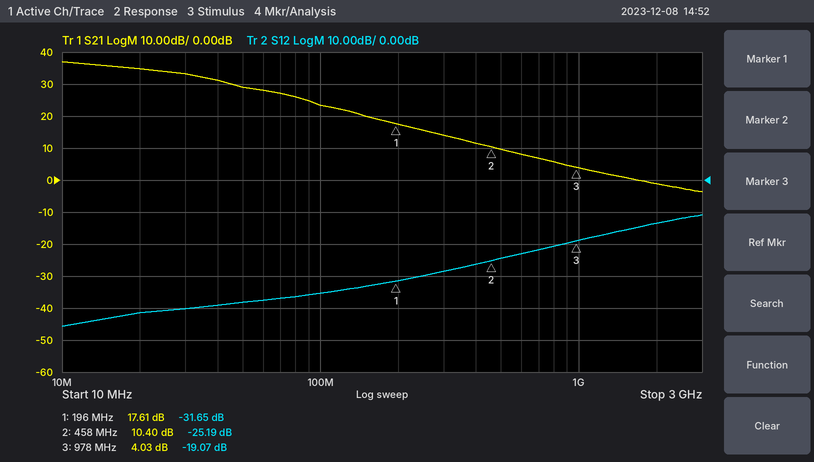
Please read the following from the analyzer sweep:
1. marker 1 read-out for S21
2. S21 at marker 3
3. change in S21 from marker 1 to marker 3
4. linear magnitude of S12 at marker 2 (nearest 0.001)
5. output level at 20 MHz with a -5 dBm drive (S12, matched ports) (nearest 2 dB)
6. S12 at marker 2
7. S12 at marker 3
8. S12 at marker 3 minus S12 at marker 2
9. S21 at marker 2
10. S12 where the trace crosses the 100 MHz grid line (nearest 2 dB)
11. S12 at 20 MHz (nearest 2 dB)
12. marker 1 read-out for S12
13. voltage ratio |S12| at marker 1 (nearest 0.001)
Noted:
17.61 dB
4.03 dB
-13.58 dB
0.055
-46 dBm
-25.19 dB
-19.07 dB
6.12 dB
10.40 dB
-36 dB
-42 dB
-31.65 dB
0.026
